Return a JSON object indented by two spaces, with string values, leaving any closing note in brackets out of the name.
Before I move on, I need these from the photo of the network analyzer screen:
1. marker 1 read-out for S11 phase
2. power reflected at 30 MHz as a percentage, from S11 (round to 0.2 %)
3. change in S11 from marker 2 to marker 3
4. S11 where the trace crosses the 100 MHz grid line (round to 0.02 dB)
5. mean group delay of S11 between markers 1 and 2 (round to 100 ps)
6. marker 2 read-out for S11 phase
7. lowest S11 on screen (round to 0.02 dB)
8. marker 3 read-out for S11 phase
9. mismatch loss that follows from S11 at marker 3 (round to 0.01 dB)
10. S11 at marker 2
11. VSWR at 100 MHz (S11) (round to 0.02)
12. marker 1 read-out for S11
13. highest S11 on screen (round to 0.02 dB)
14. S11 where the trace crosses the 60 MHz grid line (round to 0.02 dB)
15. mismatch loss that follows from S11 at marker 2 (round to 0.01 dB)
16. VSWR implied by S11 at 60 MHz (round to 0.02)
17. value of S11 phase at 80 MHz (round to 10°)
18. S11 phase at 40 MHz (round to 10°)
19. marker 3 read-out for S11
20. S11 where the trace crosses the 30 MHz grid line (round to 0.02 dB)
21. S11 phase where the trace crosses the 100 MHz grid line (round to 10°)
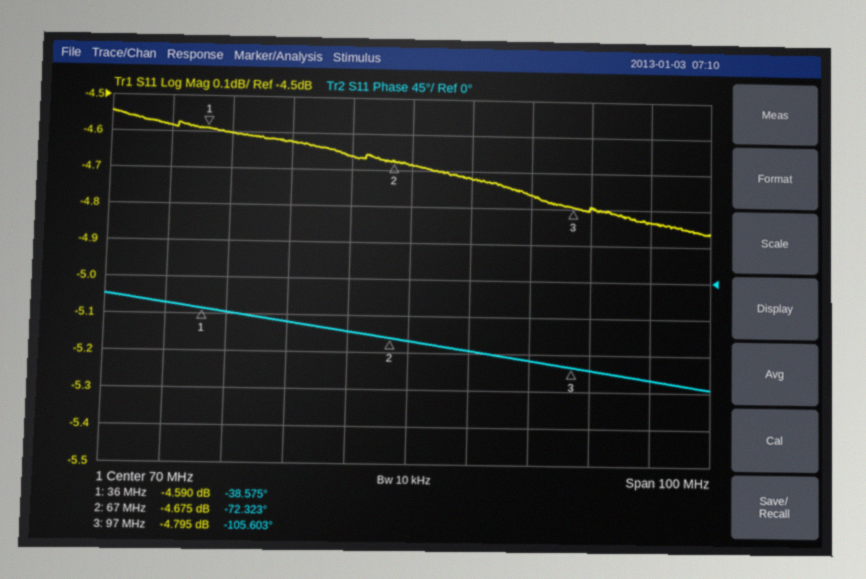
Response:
{
  "marker 1 read-out for S11 phase": "-38.575°",
  "power reflected at 30 MHz as a percentage, from S11": "34.8 %",
  "change in S11 from marker 2 to marker 3": "-0.120 dB",
  "S11 where the trace crosses the 100 MHz grid line": "-4.80 dB",
  "mean group delay of S11 between markers 1 and 2": "3.0 ns",
  "marker 2 read-out for S11 phase": "-72.323°",
  "lowest S11 on screen": "-4.86 dB",
  "marker 3 read-out for S11 phase": "-105.603°",
  "mismatch loss that follows from S11 at marker 3": "1.75 dB",
  "S11 at marker 2": "-4.675 dB",
  "VSWR at 100 MHz (S11)": "3.72",
  "marker 1 read-out for S11": "-4.590 dB",
  "highest S11 on screen": "-4.54 dB",
  "S11 where the trace crosses the 60 MHz grid line": "-4.66 dB",
  "mismatch loss that follows from S11 at marker 2": "1.81 dB",
  "VSWR implied by S11 at 60 MHz": "3.82",
  "value of S11 phase at 80 MHz": "-90°",
  "S11 phase at 40 MHz": "-40°",
  "marker 3 read-out for S11": "-4.795 dB",
  "S11 where the trace crosses the 30 MHz grid line": "-4.58 dB",
  "S11 phase where the trace crosses the 100 MHz grid line": "-110°"
}
